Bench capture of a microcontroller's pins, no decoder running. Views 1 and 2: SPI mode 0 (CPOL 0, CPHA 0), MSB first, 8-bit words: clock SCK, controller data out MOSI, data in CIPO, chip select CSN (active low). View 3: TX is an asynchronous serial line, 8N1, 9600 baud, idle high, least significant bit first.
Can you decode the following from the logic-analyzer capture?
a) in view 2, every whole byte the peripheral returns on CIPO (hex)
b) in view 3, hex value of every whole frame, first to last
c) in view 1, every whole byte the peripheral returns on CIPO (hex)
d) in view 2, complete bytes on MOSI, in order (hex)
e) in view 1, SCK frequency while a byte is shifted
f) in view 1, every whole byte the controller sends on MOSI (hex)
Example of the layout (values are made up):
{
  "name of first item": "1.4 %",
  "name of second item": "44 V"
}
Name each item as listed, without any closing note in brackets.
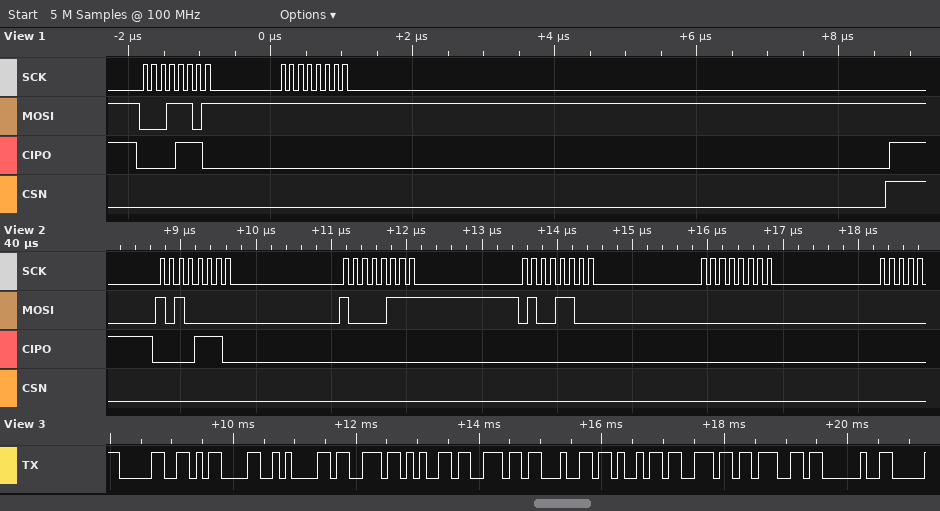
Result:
{
  "in view 2, every whole byte the peripheral returns on CIPO": "0x0E 0x00 0x00 0x00",
  "in view 3, hex value of every whole frame, first to last": "30 0D 0A 73 65 6E 64 69 6E 67 20",
  "in view 1, every whole byte the peripheral returns on CIPO": "0E 00",
  "in view 2, complete bytes on MOSI, in order": "0xA0 0x87 0x4C 0x00",
  "in view 1, SCK frequency while a byte is shifted": "8 MHz",
  "in view 1, every whole byte the controller sends on MOSI": "1D FF"
}
